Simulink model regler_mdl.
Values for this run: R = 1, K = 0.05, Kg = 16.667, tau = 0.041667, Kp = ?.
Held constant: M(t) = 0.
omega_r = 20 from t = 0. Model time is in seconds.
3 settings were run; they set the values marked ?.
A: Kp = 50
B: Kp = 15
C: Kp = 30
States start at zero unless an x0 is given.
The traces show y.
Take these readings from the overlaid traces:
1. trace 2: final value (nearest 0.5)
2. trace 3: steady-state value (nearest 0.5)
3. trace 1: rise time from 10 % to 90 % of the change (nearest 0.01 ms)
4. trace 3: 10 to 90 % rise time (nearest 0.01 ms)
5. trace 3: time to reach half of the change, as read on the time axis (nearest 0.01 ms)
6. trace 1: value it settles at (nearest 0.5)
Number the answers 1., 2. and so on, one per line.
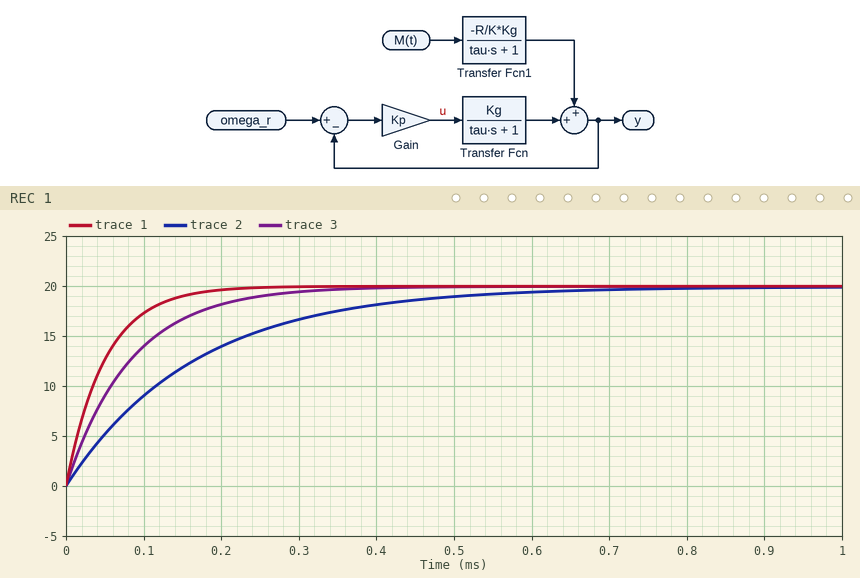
1. 20.0
2. 20.0
3. 0.11 ms
4. 0.18 ms
5. 0.06 ms
6. 20.0
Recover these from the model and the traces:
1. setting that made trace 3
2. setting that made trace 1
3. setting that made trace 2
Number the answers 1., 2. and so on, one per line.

1. C
2. A
3. B
